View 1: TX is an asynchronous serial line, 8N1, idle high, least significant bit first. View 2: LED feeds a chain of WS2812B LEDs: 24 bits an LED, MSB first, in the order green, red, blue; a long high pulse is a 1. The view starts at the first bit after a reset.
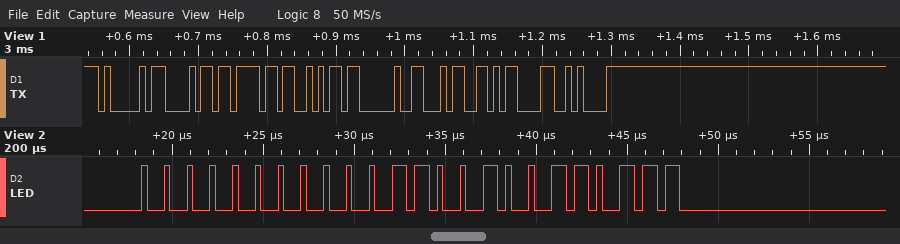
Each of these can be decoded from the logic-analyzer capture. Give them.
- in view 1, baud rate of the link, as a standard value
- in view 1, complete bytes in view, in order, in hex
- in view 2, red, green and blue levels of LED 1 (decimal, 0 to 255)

115200 baud
41 68 6F 6A 20 34 0D 0A
25, 0, 55
